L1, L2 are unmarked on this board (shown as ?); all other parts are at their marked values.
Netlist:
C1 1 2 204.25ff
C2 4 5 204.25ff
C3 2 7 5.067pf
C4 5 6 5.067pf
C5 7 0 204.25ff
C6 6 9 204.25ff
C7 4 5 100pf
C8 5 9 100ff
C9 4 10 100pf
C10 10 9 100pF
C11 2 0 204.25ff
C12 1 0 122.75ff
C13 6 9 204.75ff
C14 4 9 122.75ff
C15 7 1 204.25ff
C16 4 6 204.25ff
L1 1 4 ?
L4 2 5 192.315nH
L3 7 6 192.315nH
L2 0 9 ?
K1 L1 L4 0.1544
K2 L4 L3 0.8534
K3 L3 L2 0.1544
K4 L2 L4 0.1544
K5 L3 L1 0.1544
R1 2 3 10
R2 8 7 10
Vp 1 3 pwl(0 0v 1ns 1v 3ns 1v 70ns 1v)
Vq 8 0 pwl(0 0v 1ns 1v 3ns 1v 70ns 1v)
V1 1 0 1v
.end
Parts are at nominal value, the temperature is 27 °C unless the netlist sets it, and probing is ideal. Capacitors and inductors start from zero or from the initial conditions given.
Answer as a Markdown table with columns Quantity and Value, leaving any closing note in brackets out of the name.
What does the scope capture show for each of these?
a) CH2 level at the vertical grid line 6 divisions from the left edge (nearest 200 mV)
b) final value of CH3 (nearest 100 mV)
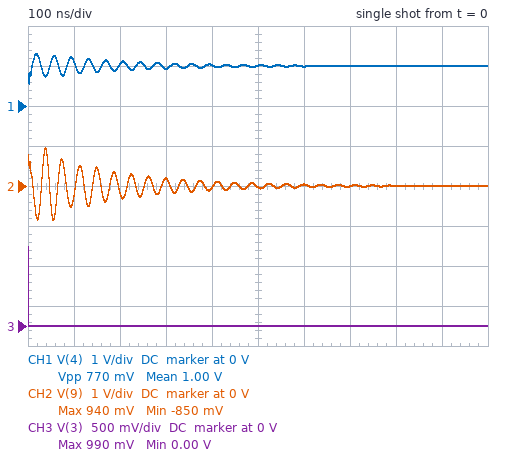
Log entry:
| Quantity | Value |
|---|---|
| CH2 level at the vertical grid line 6 divisions from the left edge | 0 V |
| final value of CH3 | 0 V |
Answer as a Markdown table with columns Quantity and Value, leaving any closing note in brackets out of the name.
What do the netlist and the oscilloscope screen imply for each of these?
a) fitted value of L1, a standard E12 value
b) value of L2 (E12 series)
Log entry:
| Quantity | Value |
|---|---|
| fitted value of L1, a standard E12 value | 100 nH |
| value of L2 | 470 nH |
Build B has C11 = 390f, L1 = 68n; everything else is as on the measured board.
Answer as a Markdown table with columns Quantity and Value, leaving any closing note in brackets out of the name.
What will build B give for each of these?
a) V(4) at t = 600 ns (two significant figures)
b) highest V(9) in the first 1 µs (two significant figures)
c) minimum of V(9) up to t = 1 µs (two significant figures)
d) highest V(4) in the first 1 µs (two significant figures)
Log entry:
| Quantity | Value |
|---|---|
| V(4) at t = 600 ns | 990 mV |
| highest V(9) in the first 1 µs | 1.0 V |
| minimum of V(9) up to t = 1 µs | -1.0 V |
| highest V(4) in the first 1 µs | 1.2 V |
